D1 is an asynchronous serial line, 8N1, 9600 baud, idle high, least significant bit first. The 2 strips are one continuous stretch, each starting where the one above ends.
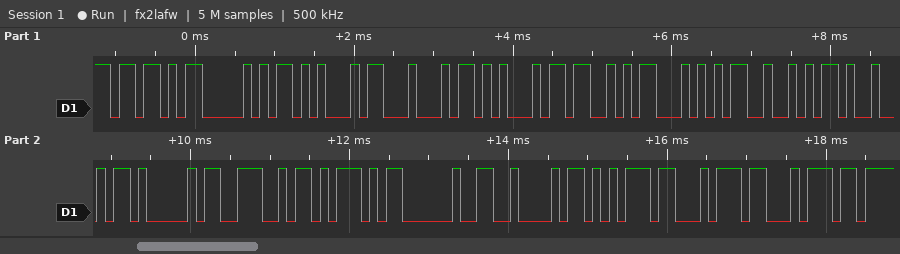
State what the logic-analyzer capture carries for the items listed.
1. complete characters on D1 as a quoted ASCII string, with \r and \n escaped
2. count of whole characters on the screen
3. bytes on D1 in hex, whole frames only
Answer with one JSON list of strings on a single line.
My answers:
["\"[PEDESTRIAN] Butt\"", "17", "0x5B 0x50 0x45 0x44 0x45 0x53 0x54 0x52 0x49 0x41 0x4E 0x5D 0x20 0x42 0x75 0x74 0x74"]
